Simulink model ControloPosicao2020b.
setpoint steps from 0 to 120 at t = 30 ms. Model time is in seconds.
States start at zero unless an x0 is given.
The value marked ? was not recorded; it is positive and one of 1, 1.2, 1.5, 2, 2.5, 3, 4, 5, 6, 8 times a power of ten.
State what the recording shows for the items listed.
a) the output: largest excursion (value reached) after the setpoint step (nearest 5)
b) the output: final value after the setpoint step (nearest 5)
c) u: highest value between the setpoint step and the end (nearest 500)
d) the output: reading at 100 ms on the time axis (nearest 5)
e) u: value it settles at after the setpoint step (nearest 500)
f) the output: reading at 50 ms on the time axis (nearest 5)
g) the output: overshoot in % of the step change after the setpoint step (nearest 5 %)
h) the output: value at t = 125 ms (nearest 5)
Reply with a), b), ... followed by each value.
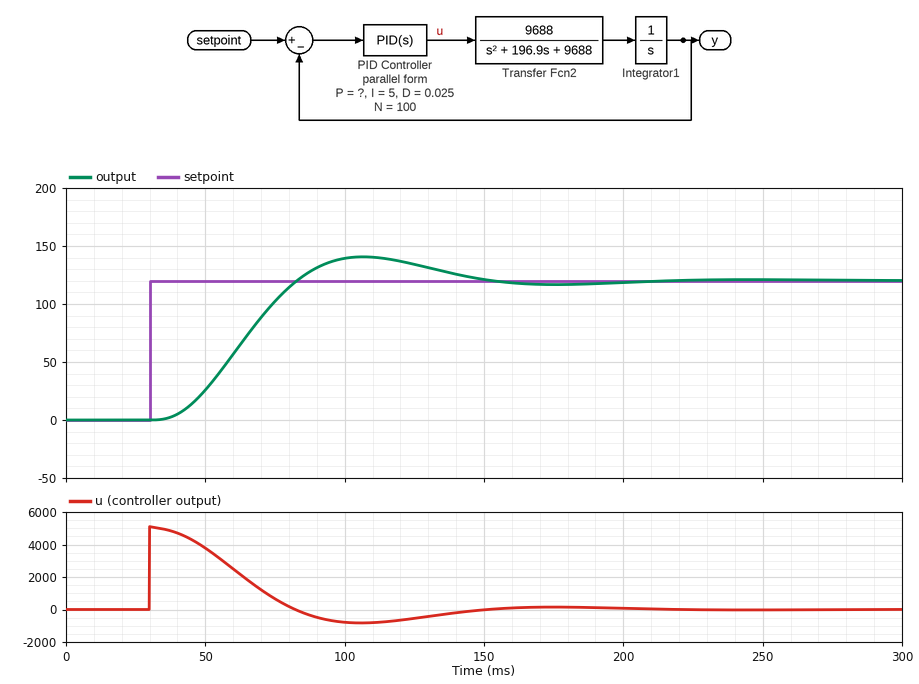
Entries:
a) 140
b) 120
c) 5000
d) 140
e) 0
f) 25
g) 15 %
h) 135
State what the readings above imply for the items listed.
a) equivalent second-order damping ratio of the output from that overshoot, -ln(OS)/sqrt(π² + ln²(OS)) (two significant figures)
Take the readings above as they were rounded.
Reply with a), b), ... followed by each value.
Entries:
a) 0.52
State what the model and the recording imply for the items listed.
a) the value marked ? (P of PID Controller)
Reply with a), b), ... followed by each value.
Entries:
a) 40
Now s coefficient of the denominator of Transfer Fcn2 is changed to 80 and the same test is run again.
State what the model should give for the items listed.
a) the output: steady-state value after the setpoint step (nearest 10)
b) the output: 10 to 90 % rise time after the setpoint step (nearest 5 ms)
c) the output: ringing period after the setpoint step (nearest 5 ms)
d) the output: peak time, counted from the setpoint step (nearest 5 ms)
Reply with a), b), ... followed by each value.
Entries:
a) 120
b) 25 ms
c) 70 ms
d) 50 ms
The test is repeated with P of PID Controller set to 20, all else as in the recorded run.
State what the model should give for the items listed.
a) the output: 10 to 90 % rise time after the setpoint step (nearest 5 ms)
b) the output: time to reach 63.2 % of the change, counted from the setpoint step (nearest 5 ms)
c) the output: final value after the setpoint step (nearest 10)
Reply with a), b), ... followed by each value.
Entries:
a) 70 ms
b) 55 ms
c) 120
